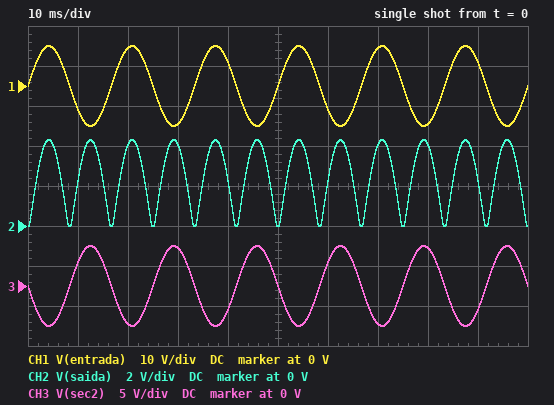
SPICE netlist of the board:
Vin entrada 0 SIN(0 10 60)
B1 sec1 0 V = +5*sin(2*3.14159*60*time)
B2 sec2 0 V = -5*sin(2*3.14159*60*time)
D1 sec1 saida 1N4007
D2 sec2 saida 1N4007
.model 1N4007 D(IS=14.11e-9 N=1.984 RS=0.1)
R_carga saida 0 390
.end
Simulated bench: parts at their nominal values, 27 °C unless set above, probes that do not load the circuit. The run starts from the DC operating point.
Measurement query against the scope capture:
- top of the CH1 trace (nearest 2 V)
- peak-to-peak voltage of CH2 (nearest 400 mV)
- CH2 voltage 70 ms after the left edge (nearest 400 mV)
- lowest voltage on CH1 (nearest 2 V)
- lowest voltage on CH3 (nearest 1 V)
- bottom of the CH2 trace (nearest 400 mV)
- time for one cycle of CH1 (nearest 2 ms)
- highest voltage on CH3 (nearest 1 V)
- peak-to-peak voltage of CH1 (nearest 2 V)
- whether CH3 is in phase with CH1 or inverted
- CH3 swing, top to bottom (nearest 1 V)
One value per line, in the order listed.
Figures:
10 V
4.4 V
4.0 V
-10 V
-5 V
0 V
16 ms
5 V
20 V
inverted
10 V
